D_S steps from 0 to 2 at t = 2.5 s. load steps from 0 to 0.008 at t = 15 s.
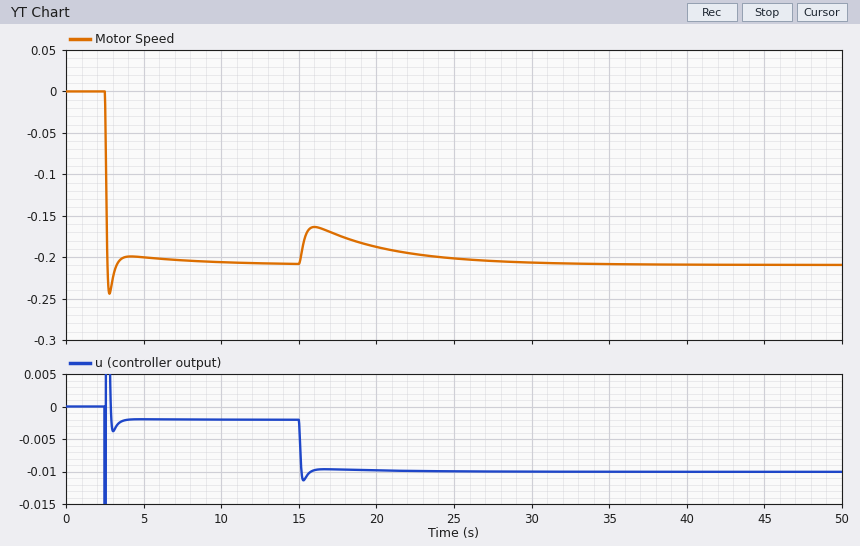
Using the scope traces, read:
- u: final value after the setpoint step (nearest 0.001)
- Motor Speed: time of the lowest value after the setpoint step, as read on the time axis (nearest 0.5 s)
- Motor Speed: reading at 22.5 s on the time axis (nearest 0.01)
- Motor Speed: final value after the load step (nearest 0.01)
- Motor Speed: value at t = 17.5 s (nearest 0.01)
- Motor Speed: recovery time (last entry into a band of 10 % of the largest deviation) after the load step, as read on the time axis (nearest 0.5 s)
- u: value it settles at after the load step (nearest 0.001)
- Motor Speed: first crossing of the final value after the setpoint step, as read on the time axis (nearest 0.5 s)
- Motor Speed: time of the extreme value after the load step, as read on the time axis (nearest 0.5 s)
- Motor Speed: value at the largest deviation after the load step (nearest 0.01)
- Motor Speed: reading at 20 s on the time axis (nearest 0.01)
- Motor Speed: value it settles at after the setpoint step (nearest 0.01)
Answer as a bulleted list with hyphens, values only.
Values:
- -0.002
- 3.0 s
- -0.20
- -0.21
- -0.17
- 28.0 s
- -0.010
- 2.5 s
- 16.0 s
- -0.16
- -0.19
- -0.21
